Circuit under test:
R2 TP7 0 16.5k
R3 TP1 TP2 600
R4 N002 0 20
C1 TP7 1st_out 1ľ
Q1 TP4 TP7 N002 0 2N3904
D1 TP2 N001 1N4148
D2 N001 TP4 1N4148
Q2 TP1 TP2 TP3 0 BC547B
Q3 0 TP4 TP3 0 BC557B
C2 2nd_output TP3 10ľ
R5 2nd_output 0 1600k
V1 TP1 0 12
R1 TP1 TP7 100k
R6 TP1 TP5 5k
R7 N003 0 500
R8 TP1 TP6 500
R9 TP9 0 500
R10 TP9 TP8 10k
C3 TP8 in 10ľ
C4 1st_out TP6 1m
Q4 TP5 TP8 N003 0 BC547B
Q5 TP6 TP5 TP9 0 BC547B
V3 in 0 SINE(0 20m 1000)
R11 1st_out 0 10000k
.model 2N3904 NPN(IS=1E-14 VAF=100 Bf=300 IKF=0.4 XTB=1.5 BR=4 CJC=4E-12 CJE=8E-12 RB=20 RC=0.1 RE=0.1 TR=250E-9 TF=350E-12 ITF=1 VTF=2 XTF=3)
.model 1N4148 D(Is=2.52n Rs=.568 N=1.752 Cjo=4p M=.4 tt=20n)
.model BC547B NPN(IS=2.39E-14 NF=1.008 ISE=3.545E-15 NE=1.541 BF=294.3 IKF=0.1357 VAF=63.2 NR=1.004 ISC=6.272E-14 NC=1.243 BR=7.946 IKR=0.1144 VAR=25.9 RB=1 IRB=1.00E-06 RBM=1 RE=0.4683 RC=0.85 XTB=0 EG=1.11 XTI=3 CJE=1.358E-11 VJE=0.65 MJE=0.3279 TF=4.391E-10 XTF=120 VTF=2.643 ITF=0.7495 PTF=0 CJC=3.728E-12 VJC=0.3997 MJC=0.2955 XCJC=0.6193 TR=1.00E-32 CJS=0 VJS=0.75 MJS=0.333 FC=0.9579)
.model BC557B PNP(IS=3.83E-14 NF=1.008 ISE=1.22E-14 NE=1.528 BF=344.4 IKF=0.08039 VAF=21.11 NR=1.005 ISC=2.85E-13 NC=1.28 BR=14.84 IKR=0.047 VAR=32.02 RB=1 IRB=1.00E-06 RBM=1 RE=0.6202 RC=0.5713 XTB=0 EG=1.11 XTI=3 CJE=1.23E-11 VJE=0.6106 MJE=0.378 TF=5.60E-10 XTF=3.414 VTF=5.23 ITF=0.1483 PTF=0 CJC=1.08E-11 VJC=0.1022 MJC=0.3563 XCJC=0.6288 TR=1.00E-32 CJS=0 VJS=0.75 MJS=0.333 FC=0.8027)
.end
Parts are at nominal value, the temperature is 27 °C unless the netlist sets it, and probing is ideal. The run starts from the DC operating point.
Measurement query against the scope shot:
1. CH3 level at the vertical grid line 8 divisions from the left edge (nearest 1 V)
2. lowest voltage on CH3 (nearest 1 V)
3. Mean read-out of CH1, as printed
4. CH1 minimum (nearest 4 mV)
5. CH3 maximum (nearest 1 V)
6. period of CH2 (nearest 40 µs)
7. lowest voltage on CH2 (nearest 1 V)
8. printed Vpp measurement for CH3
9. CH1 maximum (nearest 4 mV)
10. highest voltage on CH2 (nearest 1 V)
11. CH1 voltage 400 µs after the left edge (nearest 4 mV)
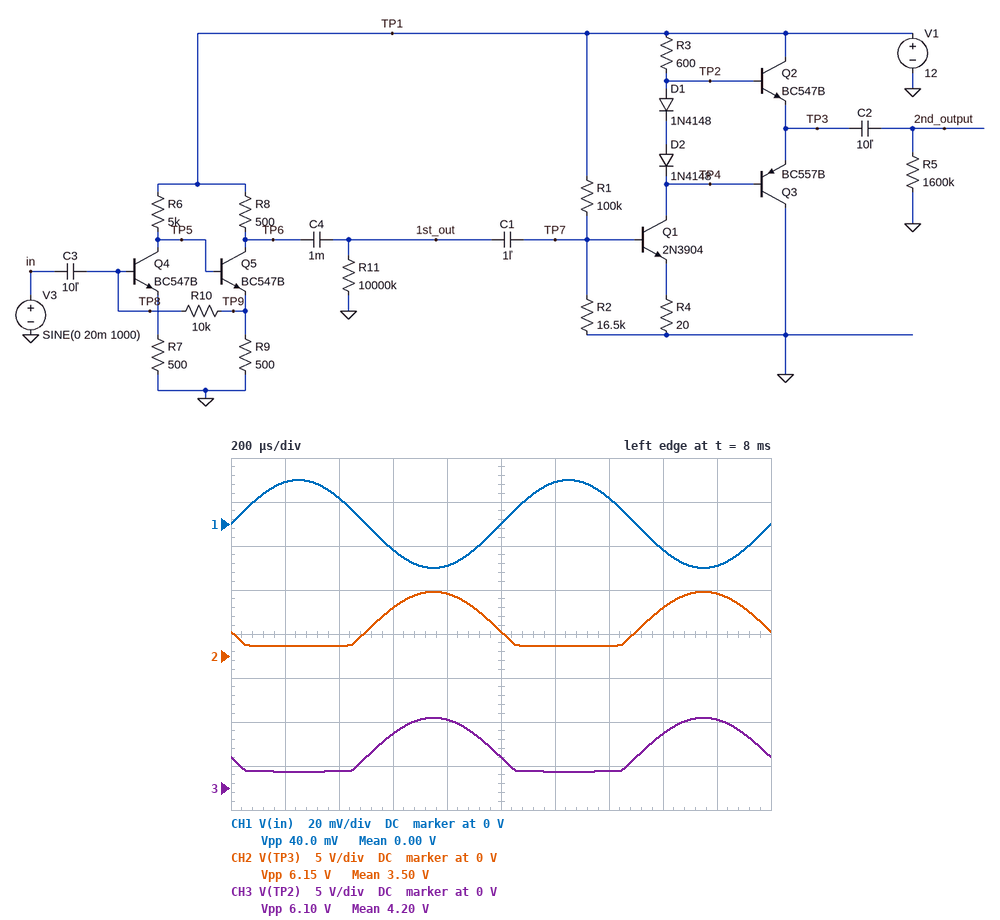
6 V
2 V
0.00 V
-20 mV
8 V
1.00 ms
1 V
6.10 V
20 mV
7 V
12 mV
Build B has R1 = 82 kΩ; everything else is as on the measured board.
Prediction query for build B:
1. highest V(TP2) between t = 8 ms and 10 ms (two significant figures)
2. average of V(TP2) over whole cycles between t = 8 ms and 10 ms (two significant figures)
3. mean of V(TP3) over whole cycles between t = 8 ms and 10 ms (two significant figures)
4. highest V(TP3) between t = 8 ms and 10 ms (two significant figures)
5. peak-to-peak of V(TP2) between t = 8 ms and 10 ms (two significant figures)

6.4 V
3.3 V
2.6 V
5.7 V
4.5 V
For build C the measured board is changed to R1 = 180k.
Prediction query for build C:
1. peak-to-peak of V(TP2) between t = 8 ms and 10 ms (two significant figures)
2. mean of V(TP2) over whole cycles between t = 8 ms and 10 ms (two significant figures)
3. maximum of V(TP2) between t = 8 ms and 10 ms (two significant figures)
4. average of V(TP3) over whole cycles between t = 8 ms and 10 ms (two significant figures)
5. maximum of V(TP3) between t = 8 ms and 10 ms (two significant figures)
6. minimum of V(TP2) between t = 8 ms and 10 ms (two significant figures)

7.1 V
8.8 V
12 V
8.2 V
11 V
4.8 V
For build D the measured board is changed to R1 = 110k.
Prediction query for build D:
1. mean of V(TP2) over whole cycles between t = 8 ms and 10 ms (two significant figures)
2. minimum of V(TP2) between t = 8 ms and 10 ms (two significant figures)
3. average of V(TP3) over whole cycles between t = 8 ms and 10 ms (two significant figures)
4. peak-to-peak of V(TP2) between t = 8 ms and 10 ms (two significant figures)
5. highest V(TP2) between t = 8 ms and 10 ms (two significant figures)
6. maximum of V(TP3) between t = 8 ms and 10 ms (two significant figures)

4.9 V
1.9 V
4.2 V
7.1 V
9.0 V
8.3 V
